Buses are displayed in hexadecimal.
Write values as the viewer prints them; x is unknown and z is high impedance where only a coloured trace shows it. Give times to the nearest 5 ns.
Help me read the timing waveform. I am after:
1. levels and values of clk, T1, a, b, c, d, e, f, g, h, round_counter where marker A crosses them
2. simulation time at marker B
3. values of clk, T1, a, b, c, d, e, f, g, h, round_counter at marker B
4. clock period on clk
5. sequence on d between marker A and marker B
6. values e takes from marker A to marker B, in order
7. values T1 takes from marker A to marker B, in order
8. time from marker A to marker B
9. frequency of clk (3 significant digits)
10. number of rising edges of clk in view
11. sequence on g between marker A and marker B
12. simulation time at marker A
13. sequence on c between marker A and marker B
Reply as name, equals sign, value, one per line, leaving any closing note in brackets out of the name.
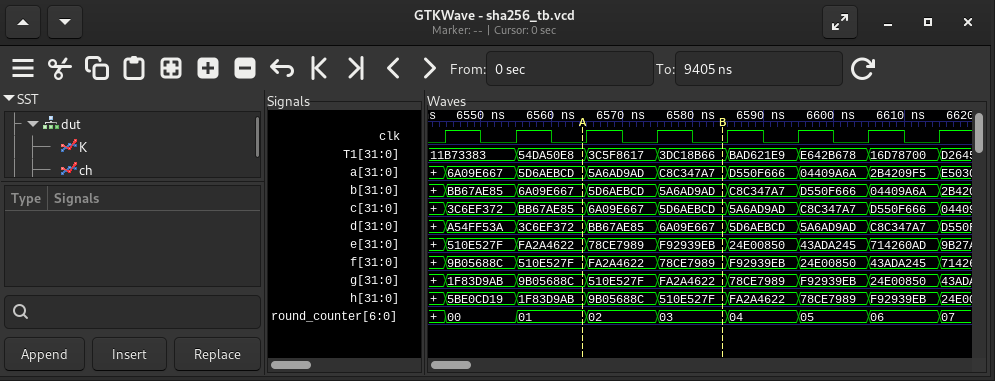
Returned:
levels and values of clk, T1, a, b, c, d, e, f, g, h, round_counter where marker A crosses them = clk=0, T1=54DA50E8, a=5D6AEBCD, b=6A09E667, c=BB67AE85, d=3C6EF372, e=FA2A4622, f=510E527F, g=9B05688C, h=1F83D9AB, round_counter=01
simulation time at marker B = 6585 ns
values of clk, T1, a, b, c, d, e, f, g, h, round_counter at marker B = clk=0, T1=3DC18B66, a=C8C347A7, b=5A6AD9AD, c=5D6AEBCD, d=6A09E667, e=F92939EB, f=78CE7989, g=FA2A4622, h=510E527F, round_counter=03
clock period on clk = 10 ns
sequence on d between marker A and marker B = 3C6EF372, BB67AE85, 6A09E667
values e takes from marker A to marker B, in order = FA2A4622, 78CE7989, F92939EB
values T1 takes from marker A to marker B, in order = 54DA50E8, 3C5F8617, 3DC18B66
time from marker A to marker B = 20 ns
frequency of clk = 100 MHz
number of rising edges of clk in view = 8
sequence on g between marker A and marker B = 9B05688C, 510E527F, FA2A4622
simulation time at marker A = 6565 ns
sequence on c between marker A and marker B = BB67AE85, 6A09E667, 5D6AEBCD
